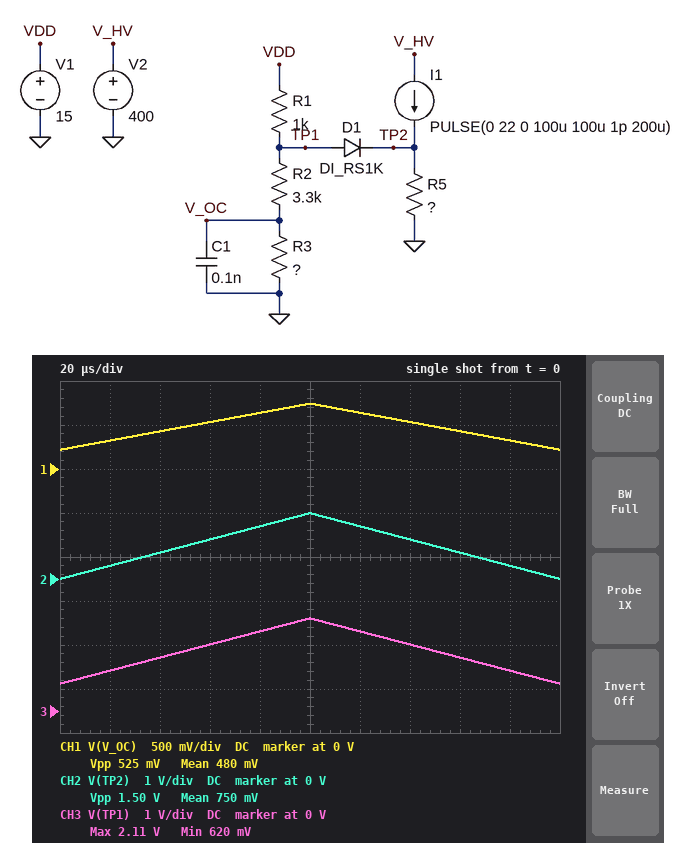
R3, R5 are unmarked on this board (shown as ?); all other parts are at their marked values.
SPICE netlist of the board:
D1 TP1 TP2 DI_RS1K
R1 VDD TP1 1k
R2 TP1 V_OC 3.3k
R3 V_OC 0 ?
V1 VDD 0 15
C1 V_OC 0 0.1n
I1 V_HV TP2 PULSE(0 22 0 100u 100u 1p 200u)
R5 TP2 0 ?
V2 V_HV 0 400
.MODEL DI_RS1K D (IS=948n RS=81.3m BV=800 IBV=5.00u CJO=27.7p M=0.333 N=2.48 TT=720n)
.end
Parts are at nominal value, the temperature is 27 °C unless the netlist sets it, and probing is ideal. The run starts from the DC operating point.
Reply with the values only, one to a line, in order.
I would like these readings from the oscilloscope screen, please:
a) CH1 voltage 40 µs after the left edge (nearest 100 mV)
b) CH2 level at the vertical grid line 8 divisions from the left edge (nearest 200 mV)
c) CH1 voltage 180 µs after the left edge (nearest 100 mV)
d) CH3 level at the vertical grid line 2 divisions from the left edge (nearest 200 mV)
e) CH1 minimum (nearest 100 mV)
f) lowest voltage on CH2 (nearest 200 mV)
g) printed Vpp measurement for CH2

400 mV
600 mV
300 mV
1.2 V
200 mV
0 V
1.50 V
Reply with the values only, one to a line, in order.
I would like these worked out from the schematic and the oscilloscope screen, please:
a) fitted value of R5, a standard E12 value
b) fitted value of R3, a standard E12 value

0.068 Ω
1.8 kΩ
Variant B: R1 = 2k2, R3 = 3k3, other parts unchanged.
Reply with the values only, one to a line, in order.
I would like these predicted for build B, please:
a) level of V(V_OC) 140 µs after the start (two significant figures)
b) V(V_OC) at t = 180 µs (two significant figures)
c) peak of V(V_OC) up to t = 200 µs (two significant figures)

730 mV
430 mV
1.0 V
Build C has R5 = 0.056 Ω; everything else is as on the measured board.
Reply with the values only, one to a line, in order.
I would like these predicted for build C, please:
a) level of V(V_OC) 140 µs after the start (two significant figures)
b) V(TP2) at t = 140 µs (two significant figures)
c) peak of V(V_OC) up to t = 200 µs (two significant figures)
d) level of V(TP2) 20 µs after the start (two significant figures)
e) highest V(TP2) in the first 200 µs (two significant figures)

480 mV
740 mV
650 mV
250 mV
1.2 V
